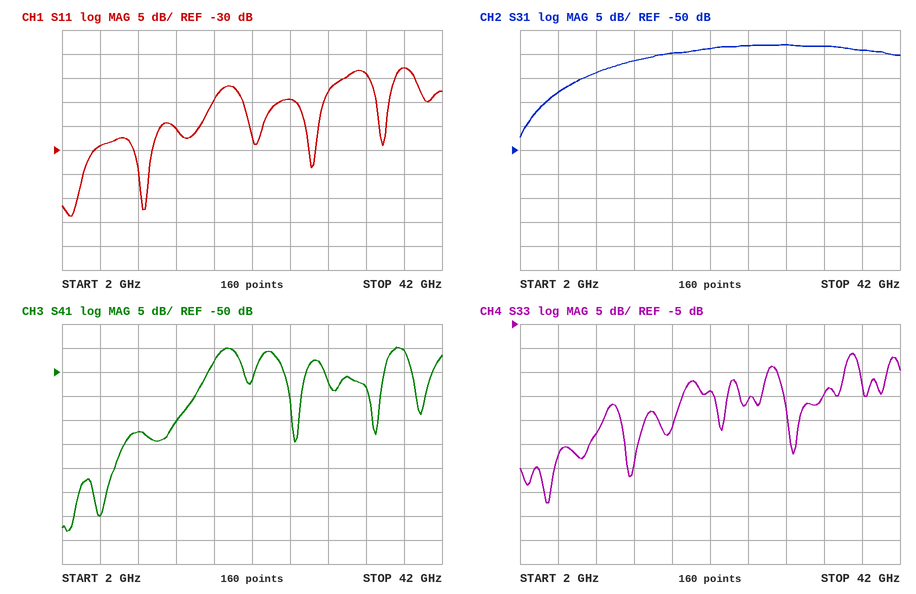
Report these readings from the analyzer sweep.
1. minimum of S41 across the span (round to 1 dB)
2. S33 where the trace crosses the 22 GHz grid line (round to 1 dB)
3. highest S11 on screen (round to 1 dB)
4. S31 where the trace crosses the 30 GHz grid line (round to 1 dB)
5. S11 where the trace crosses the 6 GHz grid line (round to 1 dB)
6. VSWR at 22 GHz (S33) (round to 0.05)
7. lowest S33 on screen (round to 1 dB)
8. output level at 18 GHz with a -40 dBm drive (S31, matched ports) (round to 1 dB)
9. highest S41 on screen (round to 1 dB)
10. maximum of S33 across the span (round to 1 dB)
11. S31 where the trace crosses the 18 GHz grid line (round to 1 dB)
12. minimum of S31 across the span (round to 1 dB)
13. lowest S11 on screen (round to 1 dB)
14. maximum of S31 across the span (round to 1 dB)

-83 dB
-19 dB
-13 dB
-28 dB
-29 dB
1.25
-42 dB
-70 dBm
-45 dB
-11 dB
-30 dB
-47 dB
-44 dB
-28 dB
